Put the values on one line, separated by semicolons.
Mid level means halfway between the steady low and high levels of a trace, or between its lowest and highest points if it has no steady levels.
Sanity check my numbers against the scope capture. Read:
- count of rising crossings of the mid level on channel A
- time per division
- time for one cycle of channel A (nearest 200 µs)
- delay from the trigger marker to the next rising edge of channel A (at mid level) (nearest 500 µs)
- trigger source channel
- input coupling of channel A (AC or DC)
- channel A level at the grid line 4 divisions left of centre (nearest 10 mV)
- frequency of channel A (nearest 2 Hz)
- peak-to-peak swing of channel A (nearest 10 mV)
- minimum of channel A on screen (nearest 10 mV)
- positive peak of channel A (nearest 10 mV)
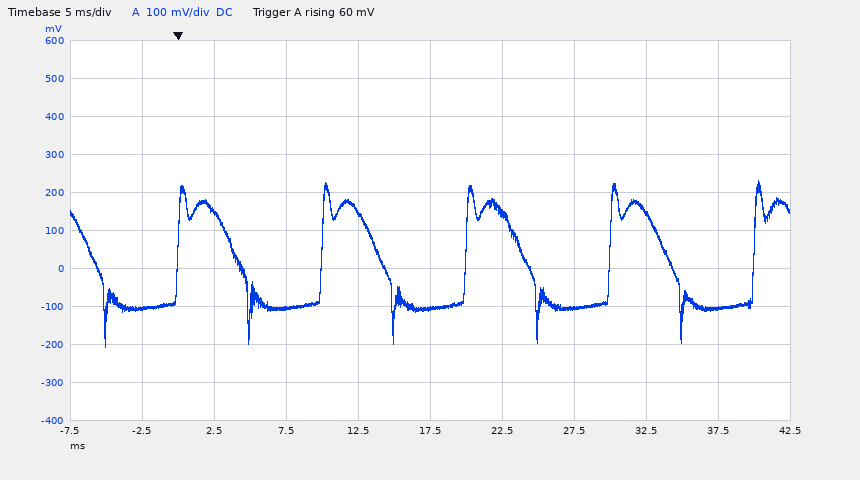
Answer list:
5; 5 ms; 10.0 ms; 10.0 ms; channel A; DC; -100 mV; 100 Hz; 440 mV; -210 mV; 230 mV
